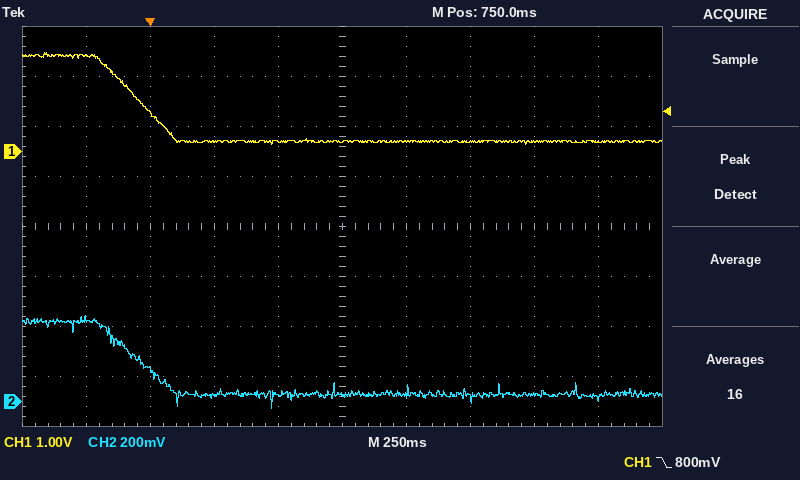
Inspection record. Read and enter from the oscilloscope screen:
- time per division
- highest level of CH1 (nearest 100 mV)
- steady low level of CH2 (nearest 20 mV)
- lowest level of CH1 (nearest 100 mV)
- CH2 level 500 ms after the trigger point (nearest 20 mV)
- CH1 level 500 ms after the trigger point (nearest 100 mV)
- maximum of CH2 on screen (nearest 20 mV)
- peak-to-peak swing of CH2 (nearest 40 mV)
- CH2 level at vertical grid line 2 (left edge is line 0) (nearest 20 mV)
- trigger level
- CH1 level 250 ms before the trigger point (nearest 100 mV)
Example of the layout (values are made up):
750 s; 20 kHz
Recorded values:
250 ms; 2.0 V; 20 mV; 100 mV; 20 mV; 200 mV; 340 mV; 360 mV; 120 mV; 800 mV; 1.9 V
